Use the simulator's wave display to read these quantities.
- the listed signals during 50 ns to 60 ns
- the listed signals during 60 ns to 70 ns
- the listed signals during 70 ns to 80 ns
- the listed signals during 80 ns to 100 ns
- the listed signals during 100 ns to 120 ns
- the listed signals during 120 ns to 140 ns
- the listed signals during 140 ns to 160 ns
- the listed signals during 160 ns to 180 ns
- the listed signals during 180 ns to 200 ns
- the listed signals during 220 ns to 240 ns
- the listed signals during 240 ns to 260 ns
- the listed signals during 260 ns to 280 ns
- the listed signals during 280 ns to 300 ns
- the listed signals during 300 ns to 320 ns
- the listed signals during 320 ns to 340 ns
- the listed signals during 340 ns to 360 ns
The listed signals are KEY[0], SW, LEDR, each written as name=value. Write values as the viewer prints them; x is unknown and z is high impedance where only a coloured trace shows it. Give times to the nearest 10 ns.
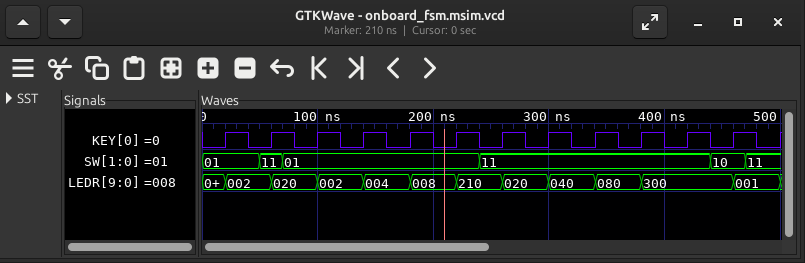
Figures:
KEY[0]=0, SW=11, LEDR=002
KEY[0]=1, SW=11, LEDR=020
KEY[0]=1, SW=01, LEDR=020
KEY[0]=0, SW=01, LEDR=020
KEY[0]=1, SW=01, LEDR=002
KEY[0]=0, SW=01, LEDR=002
KEY[0]=1, SW=01, LEDR=004
KEY[0]=0, SW=01, LEDR=004
KEY[0]=1, SW=01, LEDR=008
KEY[0]=1, SW=01, LEDR=210
KEY[0]=0, SW=11, LEDR=210
KEY[0]=1, SW=11, LEDR=020
KEY[0]=0, SW=11, LEDR=020
KEY[0]=1, SW=11, LEDR=040
KEY[0]=0, SW=11, LEDR=040
KEY[0]=1, SW=11, LEDR=080
